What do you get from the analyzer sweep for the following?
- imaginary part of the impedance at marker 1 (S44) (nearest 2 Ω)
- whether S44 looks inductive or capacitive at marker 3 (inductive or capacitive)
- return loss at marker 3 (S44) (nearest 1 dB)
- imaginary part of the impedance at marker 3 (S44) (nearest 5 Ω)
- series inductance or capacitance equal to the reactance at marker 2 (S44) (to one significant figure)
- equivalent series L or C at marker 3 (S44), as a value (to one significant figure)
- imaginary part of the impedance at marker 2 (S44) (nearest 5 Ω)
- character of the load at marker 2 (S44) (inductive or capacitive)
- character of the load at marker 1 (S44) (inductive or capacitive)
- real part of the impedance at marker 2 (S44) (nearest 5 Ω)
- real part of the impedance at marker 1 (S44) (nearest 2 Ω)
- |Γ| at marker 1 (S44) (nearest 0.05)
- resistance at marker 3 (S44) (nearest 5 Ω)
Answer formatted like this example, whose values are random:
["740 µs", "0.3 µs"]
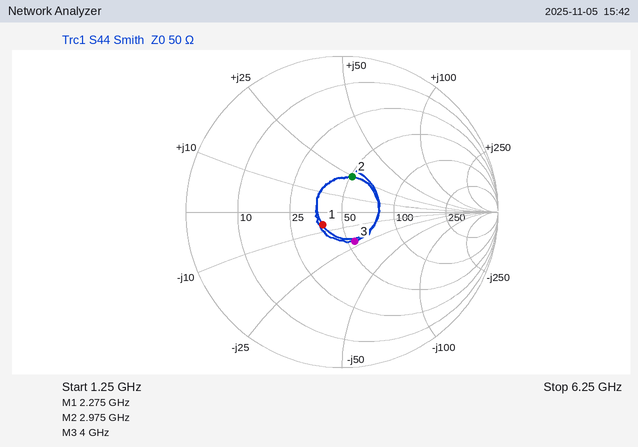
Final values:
["-6 Ω", "capacitive", "14 dB", "-20 Ω", "1 nH", "2 pF", "+25 Ω", "inductive", "capacitive", "50 Ω", "38 Ω", "0.15", "55 Ω"]
